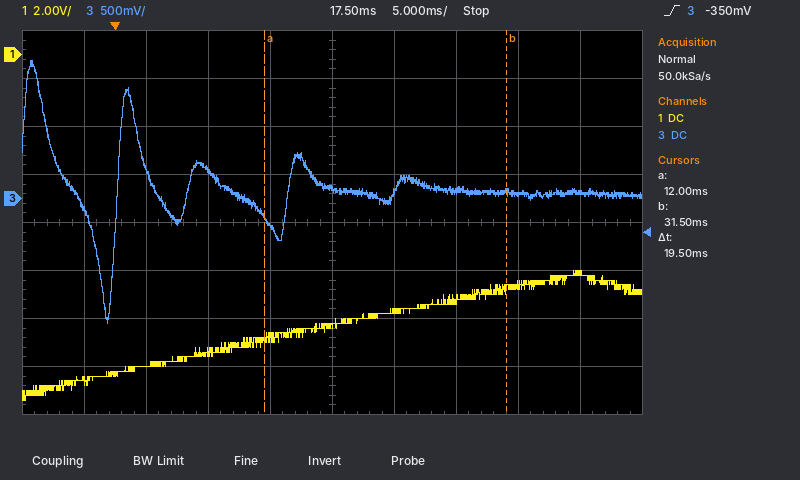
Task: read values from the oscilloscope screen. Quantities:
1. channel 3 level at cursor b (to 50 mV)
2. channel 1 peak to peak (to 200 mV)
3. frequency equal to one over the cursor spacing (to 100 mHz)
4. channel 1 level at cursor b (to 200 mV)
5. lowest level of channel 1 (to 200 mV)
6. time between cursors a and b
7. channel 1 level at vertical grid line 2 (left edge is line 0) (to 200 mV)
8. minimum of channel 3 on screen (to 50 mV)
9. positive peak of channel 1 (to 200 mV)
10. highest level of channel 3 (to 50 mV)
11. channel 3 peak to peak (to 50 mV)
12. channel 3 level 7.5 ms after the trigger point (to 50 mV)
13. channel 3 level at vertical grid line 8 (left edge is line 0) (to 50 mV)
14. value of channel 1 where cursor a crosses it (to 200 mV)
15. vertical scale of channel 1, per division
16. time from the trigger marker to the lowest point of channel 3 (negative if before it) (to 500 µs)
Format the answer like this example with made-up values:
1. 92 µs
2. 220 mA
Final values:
1. 50 mV
2. 5.4 V
3. 51.3 Hz
4. -9.8 V
5. -14.4 V
6. 19.5 ms
7. -13.0 V
8. -1.30 V
9. -9.0 V
10. 1.45 V
11. 2.75 V
12. 300 mV
13. 50 mV
14. -11.8 V
15. 2 V
16. -500 µs
